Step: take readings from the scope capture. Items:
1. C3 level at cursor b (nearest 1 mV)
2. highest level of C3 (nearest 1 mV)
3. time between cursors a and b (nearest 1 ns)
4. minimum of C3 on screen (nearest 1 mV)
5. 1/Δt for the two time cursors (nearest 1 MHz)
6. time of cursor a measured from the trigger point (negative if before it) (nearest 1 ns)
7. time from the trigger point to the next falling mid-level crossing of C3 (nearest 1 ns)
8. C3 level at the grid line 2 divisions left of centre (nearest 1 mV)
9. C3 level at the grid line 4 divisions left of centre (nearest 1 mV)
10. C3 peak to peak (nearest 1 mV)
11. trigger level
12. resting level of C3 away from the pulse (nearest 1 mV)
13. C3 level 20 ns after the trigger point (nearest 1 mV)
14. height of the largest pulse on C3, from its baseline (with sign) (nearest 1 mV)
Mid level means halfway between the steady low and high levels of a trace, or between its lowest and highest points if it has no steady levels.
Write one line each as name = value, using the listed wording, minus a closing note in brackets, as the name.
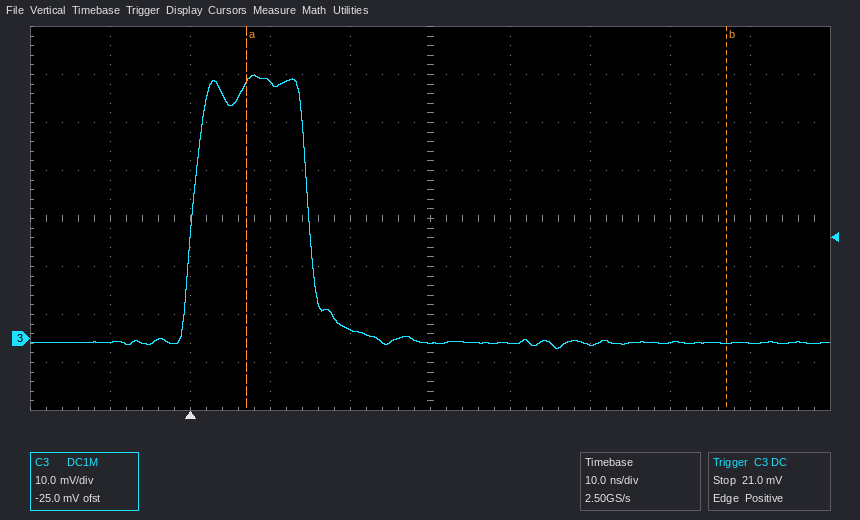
C3 level at cursor b = -1 mV
highest level of C3 = 55 mV
time between cursors a and b = 60 ns
minimum of C3 on screen = -2 mV
1/Δt for the two time cursors = 17 MHz
time of cursor a measured from the trigger point (negative if before it) = +7 ns
time from the trigger point to the next falling mid-level crossing of C3 = 15 ns
C3 level at the grid line 2 divisions left of centre = 53 mV
C3 level at the grid line 4 divisions left of centre = -1 mV
C3 peak to peak = 57 mV
trigger level = 21.0 mV
resting level of C3 away from the pulse = -1 mV
C3 level 20 ns after the trigger point = 2 mV
height of the largest pulse on C3, from its baseline (with sign) = +56 mV
